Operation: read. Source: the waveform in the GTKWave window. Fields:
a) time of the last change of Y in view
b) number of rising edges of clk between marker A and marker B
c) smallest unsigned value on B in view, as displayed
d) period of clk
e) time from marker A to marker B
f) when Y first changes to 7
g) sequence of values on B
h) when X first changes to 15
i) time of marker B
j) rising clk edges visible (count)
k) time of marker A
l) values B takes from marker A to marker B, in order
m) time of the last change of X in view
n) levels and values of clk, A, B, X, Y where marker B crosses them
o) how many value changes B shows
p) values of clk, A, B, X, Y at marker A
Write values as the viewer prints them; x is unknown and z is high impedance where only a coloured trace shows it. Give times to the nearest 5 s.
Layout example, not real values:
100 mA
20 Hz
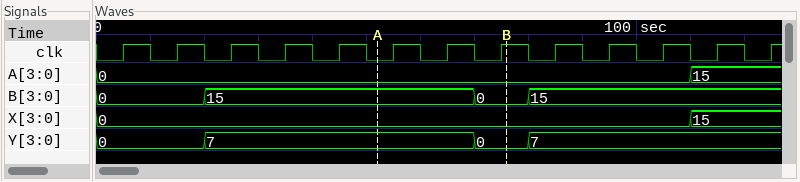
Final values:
80 s
3
0
10 s
25 s
20 s
0, 15, 0, 15
110 s
75 s
13
50 s
15, 0
110 s
clk=1, A=0, B=0, X=0, Y=0
3
clk=0, A=0, B=15, X=0, Y=7
